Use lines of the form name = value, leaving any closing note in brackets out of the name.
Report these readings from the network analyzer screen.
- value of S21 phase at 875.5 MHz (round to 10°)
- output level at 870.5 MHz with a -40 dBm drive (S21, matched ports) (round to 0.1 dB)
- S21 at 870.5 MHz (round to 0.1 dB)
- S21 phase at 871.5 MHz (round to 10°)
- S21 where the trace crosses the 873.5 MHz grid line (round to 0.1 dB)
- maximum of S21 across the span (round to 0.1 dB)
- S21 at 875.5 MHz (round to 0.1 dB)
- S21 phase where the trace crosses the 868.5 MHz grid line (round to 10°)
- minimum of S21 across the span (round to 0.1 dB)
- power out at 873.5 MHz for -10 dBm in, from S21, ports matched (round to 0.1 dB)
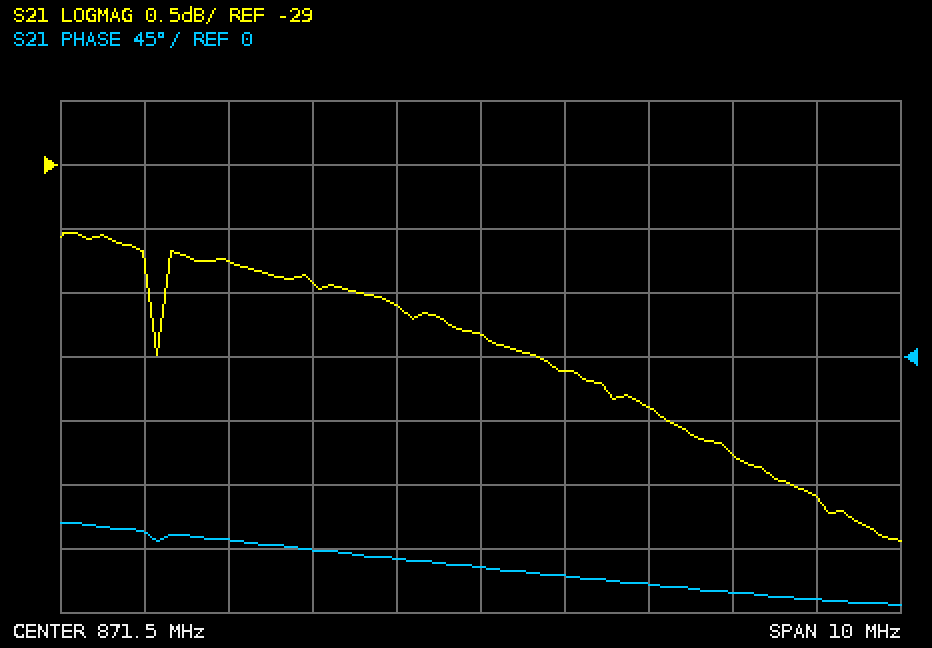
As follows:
value of S21 phase at 875.5 MHz = -170°
output level at 870.5 MHz with a -40 dBm drive (S21, matched ports) = -70.1 dBm
S21 at 870.5 MHz = -30.1 dB
S21 phase at 871.5 MHz = -150°
S21 where the trace crosses the 873.5 MHz grid line = -30.9 dB
maximum of S21 across the span = -29.5 dB
S21 at 875.5 MHz = -31.6 dB
S21 phase where the trace crosses the 868.5 MHz grid line = -130°
minimum of S21 across the span = -31.9 dB
power out at 873.5 MHz for -10 dBm in, from S21, ports matched = -40.9 dBm
